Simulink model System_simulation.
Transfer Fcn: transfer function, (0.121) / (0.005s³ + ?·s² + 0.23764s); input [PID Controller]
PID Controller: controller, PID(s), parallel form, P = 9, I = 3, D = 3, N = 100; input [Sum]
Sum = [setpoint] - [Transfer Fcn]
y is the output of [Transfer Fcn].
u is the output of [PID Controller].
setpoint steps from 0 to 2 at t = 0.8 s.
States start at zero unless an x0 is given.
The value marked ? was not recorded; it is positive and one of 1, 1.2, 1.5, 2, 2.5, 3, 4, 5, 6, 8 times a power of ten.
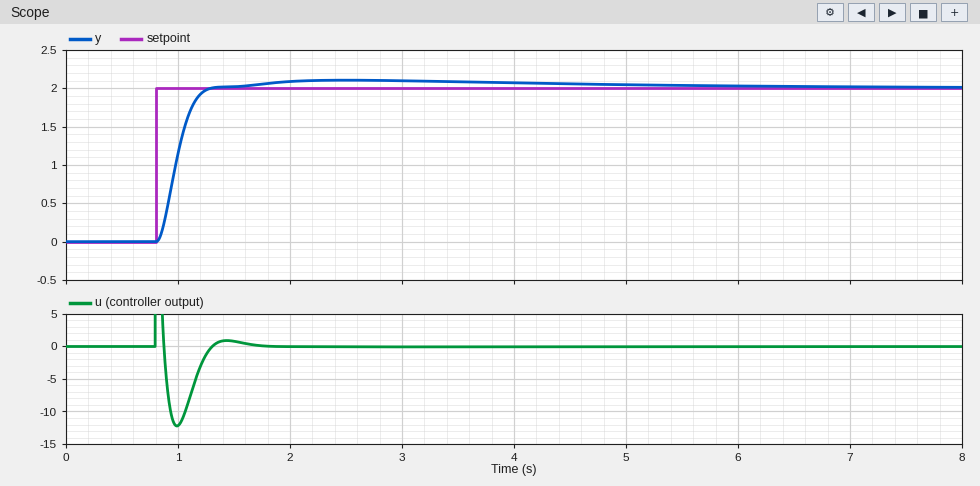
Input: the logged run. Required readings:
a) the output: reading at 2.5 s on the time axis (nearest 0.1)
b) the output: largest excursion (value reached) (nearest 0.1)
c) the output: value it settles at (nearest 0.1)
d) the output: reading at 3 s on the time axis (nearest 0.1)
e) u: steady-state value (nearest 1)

2.1
2.1
2.0
2.1
0
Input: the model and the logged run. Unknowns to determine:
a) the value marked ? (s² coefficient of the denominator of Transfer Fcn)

0.08
